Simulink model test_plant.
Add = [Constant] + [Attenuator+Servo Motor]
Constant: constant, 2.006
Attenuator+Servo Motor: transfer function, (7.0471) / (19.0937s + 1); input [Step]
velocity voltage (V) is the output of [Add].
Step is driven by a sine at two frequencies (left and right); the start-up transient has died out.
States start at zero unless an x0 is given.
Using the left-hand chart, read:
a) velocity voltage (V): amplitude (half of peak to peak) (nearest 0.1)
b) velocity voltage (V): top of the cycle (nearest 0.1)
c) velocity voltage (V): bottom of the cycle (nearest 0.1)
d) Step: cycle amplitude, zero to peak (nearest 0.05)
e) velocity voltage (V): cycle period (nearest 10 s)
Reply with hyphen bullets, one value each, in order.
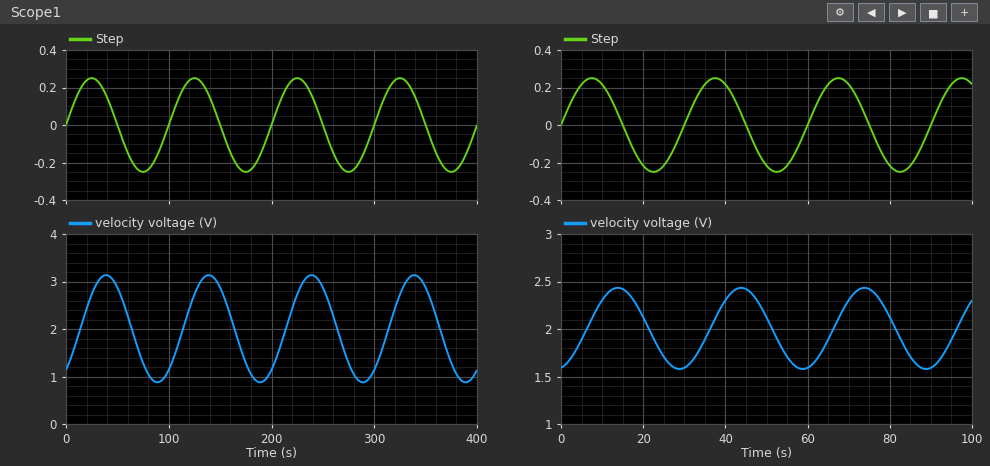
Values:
- 1.1
- 3.1
- 0.9
- 0.25
- 100 s
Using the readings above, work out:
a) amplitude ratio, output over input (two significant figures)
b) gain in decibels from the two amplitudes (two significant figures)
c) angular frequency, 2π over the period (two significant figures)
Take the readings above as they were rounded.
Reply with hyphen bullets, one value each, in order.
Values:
- 4.4
- 13 dB
- 0.063 rad/s
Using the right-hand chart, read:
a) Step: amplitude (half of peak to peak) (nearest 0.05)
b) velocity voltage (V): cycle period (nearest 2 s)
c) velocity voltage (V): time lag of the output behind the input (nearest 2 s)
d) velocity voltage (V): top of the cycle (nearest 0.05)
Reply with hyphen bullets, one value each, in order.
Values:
- 0.25
- 30 s
- 6 s
- 2.45
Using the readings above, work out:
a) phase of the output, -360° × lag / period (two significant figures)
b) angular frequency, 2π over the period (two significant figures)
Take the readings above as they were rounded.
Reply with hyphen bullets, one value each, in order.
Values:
- -72°
- 0.21 rad/s
